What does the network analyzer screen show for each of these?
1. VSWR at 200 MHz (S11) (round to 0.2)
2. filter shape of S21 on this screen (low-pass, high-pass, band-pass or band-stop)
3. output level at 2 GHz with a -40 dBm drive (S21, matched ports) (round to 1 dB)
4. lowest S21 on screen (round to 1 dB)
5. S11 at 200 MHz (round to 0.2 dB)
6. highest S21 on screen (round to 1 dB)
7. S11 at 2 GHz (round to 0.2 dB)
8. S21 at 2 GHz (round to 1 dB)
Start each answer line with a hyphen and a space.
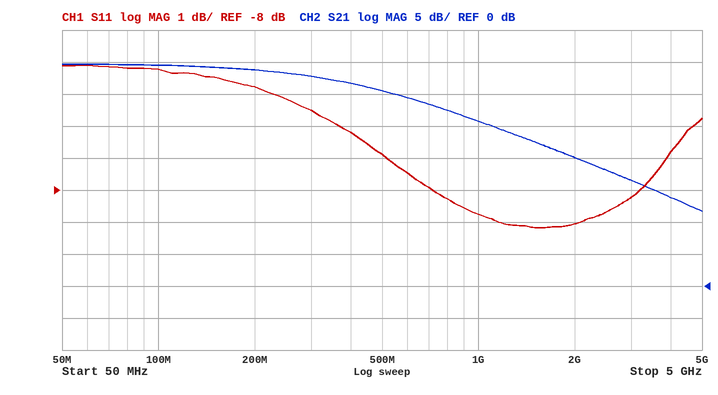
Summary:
- 3.8
- low-pass
- -20 dBm
- 12 dB
- -4.8 dB
- 35 dB
- -9.0 dB
- 20 dB
